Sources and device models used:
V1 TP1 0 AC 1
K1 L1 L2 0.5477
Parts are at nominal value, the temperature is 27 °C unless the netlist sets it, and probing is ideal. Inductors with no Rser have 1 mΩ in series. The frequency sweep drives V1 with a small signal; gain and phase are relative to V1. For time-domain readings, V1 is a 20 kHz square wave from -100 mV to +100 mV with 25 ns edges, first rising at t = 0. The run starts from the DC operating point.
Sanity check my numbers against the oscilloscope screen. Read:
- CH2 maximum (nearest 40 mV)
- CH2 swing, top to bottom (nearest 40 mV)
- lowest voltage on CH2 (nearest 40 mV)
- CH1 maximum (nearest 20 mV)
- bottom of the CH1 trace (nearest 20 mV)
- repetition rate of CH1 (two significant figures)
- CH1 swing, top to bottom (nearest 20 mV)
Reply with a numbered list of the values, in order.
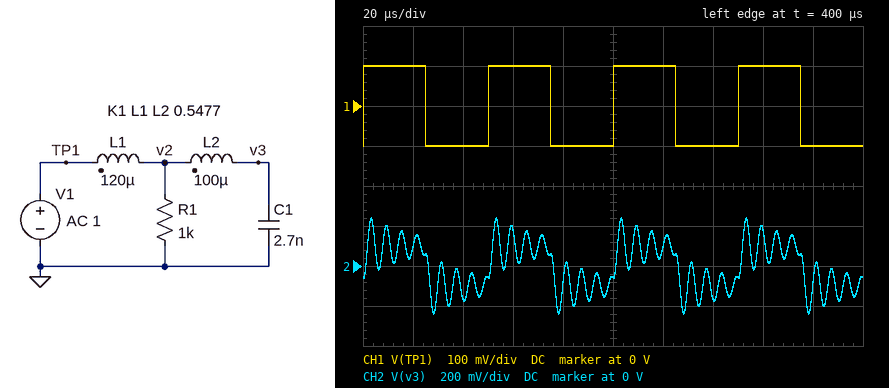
1. 240 mV
2. 480 mV
3. -240 mV
4. 100 mV
5. -100 mV
6. 20 kHz
7. 200 mV
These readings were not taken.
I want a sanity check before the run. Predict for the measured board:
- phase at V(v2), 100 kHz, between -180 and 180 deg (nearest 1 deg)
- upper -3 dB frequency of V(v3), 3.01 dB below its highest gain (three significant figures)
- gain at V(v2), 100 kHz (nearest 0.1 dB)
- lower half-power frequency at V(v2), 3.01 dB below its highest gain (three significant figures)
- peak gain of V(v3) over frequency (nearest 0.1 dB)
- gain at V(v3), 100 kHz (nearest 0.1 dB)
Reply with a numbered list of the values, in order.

1. -6 deg
2. 174 kHz
3. 2.2 dB
4. 156 kHz
5. 20.1 dB
6. 3.9 dB
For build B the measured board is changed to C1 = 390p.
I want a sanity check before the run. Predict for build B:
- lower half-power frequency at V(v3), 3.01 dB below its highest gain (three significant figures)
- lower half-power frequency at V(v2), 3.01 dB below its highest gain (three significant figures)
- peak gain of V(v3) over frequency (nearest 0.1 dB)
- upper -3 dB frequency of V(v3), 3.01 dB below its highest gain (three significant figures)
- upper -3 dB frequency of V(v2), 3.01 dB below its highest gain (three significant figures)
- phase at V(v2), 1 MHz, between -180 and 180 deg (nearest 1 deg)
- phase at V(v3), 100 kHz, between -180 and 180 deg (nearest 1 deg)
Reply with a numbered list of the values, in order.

1. 371 kHz
2. 326 kHz
3. 11.8 dB
4. 489 kHz
5. 468 kHz
6. -1 deg
7. -7 deg
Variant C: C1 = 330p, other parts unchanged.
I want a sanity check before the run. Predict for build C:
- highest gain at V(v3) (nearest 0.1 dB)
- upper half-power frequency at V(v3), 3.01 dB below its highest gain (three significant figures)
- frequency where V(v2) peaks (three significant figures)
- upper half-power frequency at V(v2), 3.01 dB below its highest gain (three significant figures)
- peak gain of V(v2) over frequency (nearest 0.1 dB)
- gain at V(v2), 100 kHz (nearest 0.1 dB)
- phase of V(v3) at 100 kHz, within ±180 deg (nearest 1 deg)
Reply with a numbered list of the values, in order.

1. 11.1 dB
2. 536 kHz
3. 452 kHz
4. 510 kHz
5. 5.8 dB
6. 0.2 dB
7. -7 deg
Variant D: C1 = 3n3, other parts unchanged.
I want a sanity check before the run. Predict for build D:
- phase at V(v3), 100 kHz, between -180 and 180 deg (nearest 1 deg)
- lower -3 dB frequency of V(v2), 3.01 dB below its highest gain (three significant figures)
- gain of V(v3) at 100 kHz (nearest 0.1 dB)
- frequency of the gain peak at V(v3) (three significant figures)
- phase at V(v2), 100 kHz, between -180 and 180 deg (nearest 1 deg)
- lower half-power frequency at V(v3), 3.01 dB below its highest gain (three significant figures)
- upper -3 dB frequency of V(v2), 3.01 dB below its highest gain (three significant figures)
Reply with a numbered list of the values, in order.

1. -9 deg
2. 142 kHz
3. 5.0 dB
4. 150 kHz
5. -7 deg
6. 143 kHz
7. 156 kHz
